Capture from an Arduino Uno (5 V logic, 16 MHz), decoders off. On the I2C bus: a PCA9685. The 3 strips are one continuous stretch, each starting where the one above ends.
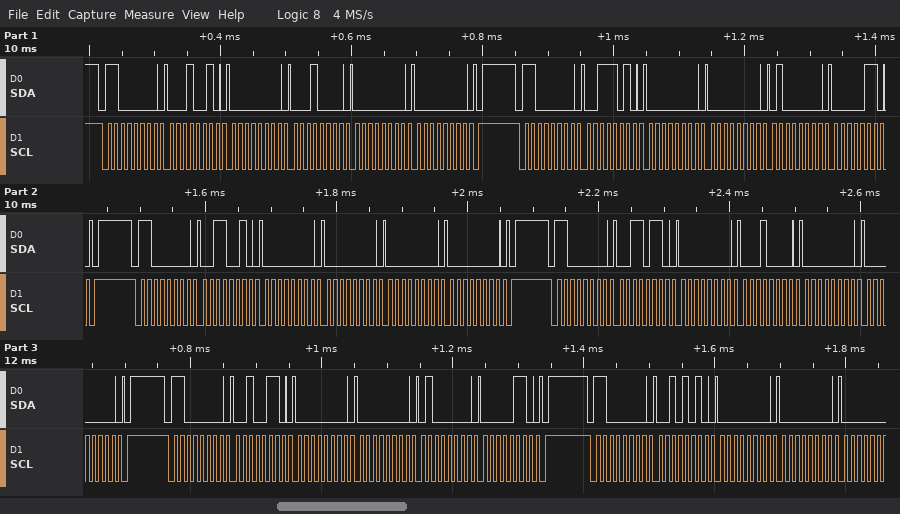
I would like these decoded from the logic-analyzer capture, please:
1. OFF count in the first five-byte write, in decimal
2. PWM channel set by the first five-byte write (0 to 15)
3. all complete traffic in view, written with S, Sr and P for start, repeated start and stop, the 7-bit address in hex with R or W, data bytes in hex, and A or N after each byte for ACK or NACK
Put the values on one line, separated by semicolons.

0; 3; S 60W A 12 A 00 A 10 A 00 A 00 A P S 60W A 3A A 00 A 00 A 40 A 06 A P S 60W A 32 A 00 A 00 A 00 A 00 A P S 60W A 36 A 00 A 10 A 00 A 00 A P S 60W A 26 A 00 A 00 A 40 A 06 A P S 60W A 2A A 00 A 00 A
